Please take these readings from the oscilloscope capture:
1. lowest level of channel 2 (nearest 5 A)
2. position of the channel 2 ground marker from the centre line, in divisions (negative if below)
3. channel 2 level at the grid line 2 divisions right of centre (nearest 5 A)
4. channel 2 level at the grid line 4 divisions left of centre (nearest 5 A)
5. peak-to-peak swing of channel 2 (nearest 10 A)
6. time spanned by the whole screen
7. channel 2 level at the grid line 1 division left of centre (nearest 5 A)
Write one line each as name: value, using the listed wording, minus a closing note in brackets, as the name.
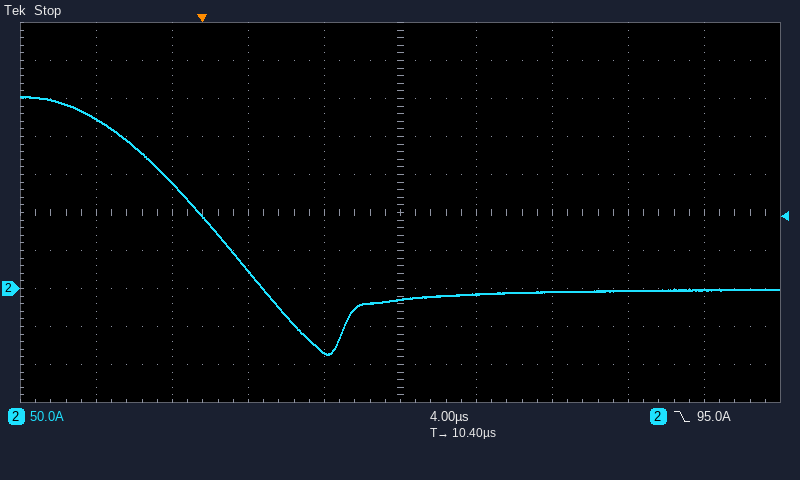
lowest level of channel 2: -85 A
position of the channel 2 ground marker from the centre line, in divisions: -2.0 div
channel 2 level at the grid line 2 divisions right of centre: -5 A
channel 2 level at the grid line 4 divisions left of centre: 225 A
peak-to-peak swing of channel 2: 340 A
time spanned by the whole screen: 40 µs
channel 2 level at the grid line 1 division left of centre: -85 A
